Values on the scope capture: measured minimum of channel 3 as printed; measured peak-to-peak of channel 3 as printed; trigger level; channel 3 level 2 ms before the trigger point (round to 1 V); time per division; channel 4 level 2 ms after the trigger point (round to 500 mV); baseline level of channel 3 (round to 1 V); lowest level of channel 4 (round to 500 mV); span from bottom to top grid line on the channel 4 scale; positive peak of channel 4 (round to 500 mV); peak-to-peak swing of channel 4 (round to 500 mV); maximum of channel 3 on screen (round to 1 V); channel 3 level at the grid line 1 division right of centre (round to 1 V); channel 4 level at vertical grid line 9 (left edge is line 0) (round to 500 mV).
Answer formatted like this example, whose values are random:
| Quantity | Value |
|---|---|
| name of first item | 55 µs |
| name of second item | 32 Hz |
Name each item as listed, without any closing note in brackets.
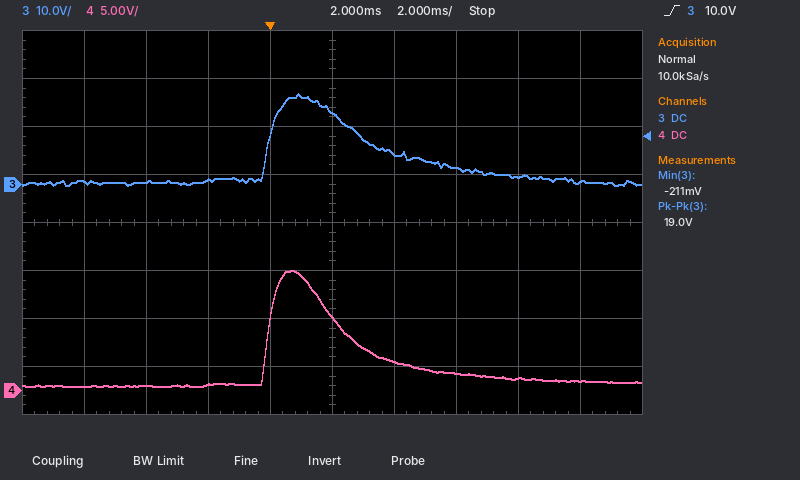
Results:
| Quantity | Value |
|---|---|
| measured minimum of channel 3 as printed | -211 mV |
| measured peak-to-peak of channel 3 as printed | 19.0 V |
| trigger level | 10.0 V |
| channel 3 level 2 ms before the trigger point | 1 V |
| time per division | 2 ms |
| channel 4 level 2 ms after the trigger point | 7.5 V |
| baseline level of channel 3 | 0 V |
| lowest level of channel 4 | 500 mV |
| span from bottom to top grid line on the channel 4 scale | 40 V |
| positive peak of channel 4 | 12.5 V |
| peak-to-peak swing of channel 4 | 12.0 V |
| maximum of channel 3 on screen | 19 V |
| channel 3 level at the grid line 1 division right of centre | 6 V |
| channel 4 level at vertical grid line 9 (left edge is line 0) | 1.0 V |
